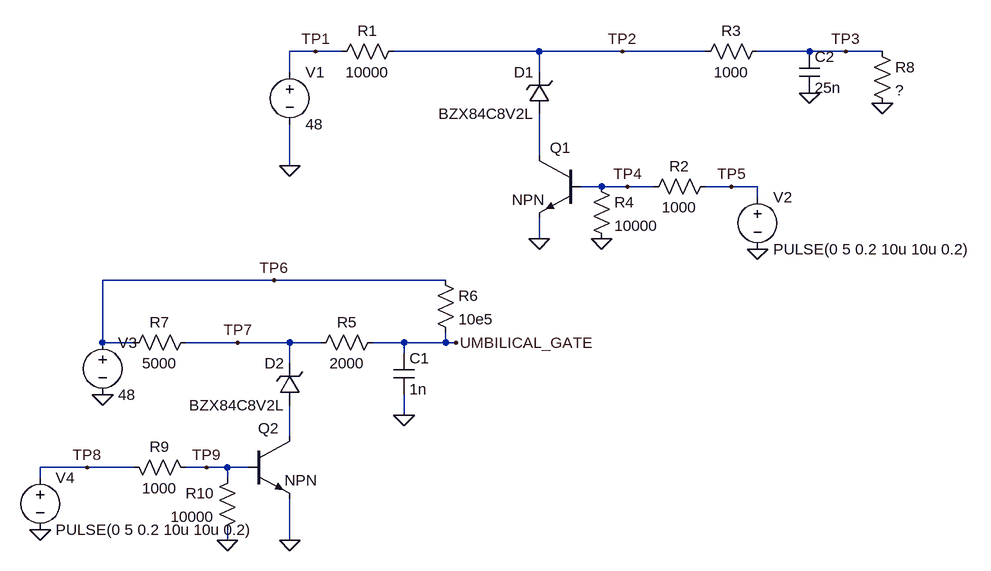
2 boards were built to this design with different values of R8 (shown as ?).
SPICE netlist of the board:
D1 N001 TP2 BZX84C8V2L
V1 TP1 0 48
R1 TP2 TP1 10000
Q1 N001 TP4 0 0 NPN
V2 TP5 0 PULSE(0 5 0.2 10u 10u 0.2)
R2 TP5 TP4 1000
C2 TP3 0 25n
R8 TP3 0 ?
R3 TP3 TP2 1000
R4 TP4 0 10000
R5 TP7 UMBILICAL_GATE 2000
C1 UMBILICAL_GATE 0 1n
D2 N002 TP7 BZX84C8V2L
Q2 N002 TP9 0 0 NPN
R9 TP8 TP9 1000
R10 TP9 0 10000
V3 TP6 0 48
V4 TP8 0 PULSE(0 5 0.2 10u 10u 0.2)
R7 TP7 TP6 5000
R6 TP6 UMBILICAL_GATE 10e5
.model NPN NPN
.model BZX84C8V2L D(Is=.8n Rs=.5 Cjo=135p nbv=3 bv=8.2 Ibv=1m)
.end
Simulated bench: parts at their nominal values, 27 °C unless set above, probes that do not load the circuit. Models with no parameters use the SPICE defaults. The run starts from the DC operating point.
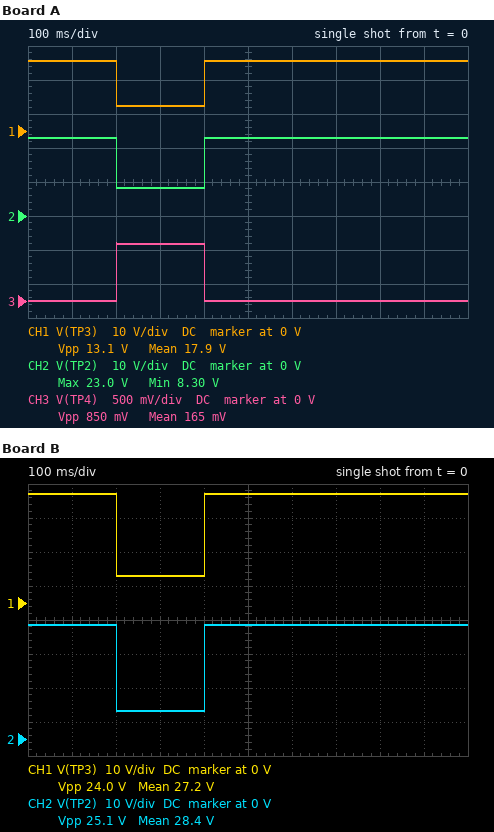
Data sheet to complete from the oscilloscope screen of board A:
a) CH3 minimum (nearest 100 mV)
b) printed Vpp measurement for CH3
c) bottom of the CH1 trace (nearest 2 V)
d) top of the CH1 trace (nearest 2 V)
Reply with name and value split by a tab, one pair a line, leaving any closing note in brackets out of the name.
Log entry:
CH3 minimum	0 V
printed Vpp measurement for CH3	850 mV
bottom of the CH1 trace	8 V
top of the CH1 trace	20 V
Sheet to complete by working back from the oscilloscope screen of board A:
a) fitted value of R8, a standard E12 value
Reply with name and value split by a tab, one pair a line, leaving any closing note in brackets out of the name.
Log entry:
fitted value of R8, a standard E12 value	8.2 kΩ
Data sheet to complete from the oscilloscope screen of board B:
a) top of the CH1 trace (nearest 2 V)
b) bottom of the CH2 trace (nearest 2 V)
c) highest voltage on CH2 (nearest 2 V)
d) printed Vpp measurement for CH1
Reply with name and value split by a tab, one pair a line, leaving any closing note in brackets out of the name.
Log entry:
top of the CH1 trace	32 V
bottom of the CH2 trace	8 V
highest voltage on CH2	34 V
printed Vpp measurement for CH1	24.0 V
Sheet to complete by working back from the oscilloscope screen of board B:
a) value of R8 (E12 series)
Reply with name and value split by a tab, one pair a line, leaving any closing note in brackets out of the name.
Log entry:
value of R8	22 kΩ
